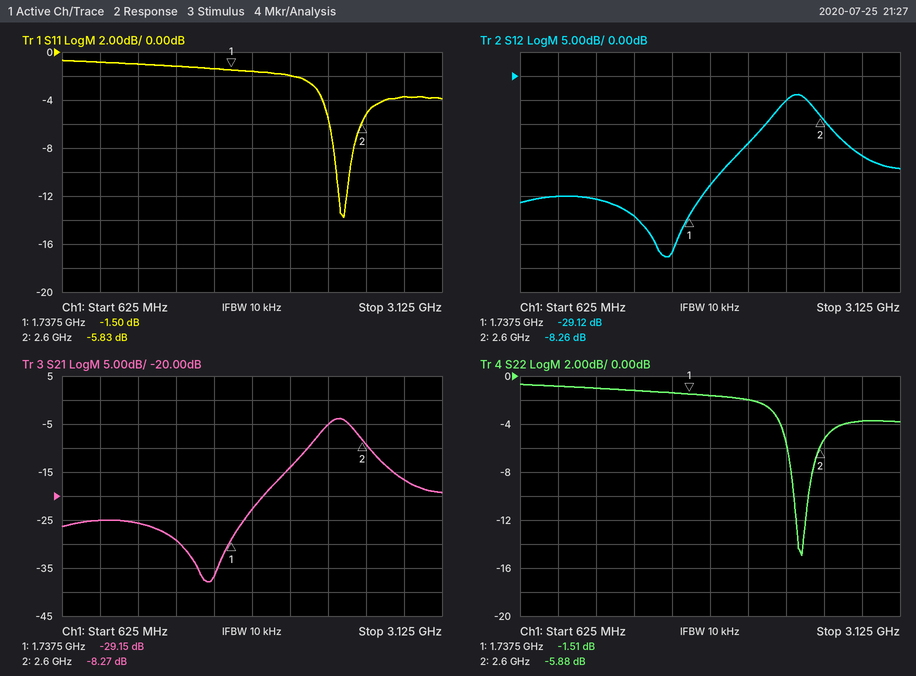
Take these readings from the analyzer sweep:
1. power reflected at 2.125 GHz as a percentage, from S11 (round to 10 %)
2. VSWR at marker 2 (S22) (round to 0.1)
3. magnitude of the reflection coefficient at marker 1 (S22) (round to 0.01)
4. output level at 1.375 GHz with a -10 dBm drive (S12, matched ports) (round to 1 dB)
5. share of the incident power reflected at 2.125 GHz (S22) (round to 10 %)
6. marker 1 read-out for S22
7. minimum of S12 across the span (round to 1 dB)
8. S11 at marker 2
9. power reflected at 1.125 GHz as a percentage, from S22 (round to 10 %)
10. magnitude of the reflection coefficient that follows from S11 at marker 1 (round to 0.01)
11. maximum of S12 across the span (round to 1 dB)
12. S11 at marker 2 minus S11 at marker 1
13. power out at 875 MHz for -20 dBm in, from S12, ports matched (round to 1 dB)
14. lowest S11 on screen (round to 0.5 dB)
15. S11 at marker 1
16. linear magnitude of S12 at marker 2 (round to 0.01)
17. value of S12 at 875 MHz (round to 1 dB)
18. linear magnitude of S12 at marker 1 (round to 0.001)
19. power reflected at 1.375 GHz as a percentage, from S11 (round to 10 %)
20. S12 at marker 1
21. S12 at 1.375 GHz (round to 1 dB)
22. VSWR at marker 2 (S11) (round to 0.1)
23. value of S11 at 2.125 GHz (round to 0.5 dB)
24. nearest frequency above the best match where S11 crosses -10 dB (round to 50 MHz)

60 %
3.1
0.84
-39 dBm
60 %
-1.51 dB
-38 dB
-5.83 dB
80 %
0.84
-4 dB
-4.33 dB
-45 dBm
-14.0 dB
-1.50 dB
0.39
-25 dB
0.035
80 %
-29.12 dB
-29 dB
3.1
-2.0 dB
2.50 GHz
